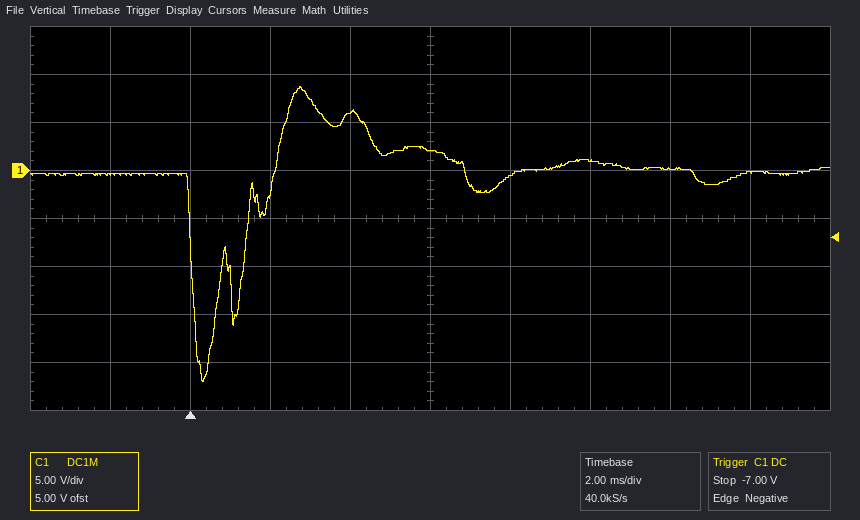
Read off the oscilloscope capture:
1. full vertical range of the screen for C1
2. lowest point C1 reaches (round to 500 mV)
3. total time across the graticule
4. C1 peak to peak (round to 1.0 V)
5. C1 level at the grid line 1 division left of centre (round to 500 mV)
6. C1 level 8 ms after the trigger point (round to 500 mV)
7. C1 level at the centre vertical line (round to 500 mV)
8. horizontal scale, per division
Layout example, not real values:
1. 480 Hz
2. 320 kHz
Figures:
1. 40 V
2. -22.0 V
3. 20 ms
4. 31.0 V
5. 6.0 V
6. -500 mV
7. 2.0 V
8. 2 ms
